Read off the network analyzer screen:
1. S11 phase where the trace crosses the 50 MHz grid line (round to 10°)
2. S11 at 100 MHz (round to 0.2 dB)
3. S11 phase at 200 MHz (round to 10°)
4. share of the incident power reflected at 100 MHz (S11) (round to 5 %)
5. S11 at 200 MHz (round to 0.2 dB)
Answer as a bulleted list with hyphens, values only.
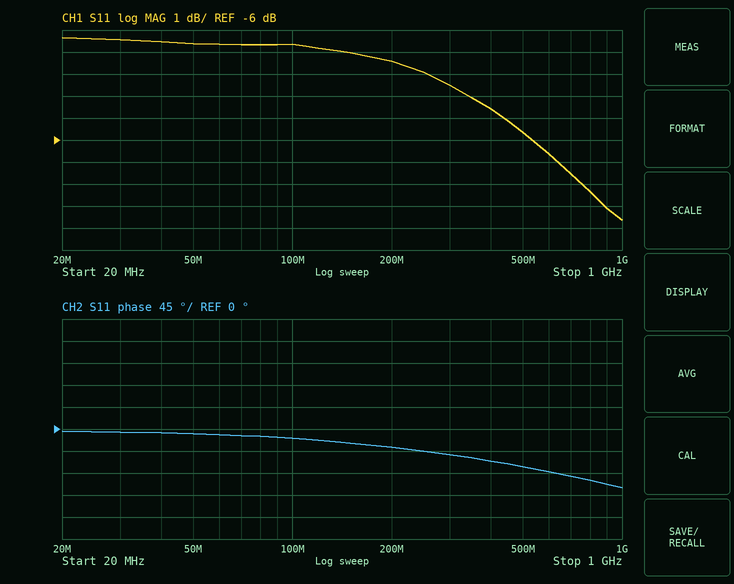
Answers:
- -10°
- -1.6 dB
- -40°
- 70 %
- -2.4 dB
